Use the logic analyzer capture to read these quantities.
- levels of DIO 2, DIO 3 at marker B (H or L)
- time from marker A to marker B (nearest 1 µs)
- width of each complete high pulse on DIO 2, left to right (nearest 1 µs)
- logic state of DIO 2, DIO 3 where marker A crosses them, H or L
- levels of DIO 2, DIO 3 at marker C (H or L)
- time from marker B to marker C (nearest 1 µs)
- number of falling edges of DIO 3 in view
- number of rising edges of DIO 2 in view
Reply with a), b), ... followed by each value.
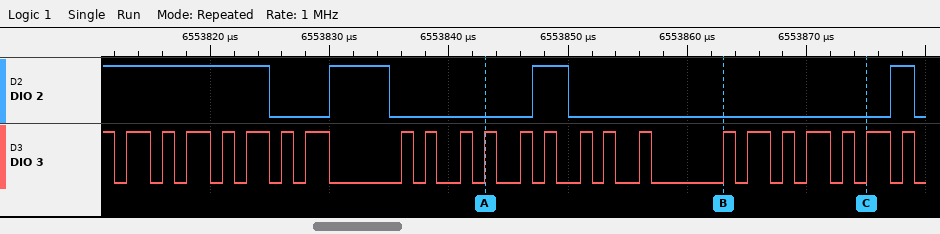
a) DIO 2=L, DIO 3=H
b) 20 µs
c) 5 µs, 3 µs, 2 µs
d) DIO 2=L, DIO 3=H
e) DIO 2=L, DIO 3=H
f) 12 µs
g) 24
h) 3
